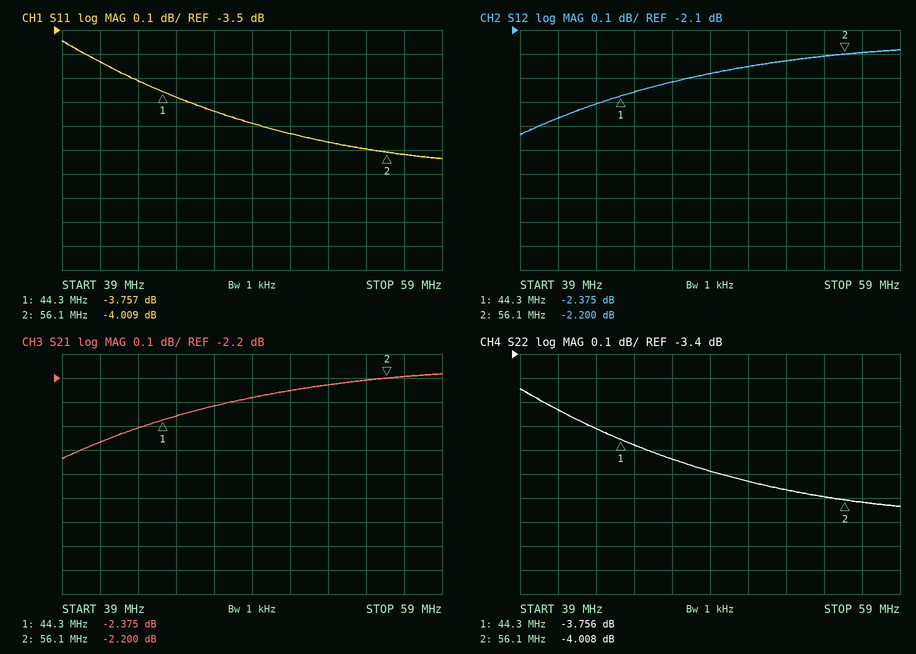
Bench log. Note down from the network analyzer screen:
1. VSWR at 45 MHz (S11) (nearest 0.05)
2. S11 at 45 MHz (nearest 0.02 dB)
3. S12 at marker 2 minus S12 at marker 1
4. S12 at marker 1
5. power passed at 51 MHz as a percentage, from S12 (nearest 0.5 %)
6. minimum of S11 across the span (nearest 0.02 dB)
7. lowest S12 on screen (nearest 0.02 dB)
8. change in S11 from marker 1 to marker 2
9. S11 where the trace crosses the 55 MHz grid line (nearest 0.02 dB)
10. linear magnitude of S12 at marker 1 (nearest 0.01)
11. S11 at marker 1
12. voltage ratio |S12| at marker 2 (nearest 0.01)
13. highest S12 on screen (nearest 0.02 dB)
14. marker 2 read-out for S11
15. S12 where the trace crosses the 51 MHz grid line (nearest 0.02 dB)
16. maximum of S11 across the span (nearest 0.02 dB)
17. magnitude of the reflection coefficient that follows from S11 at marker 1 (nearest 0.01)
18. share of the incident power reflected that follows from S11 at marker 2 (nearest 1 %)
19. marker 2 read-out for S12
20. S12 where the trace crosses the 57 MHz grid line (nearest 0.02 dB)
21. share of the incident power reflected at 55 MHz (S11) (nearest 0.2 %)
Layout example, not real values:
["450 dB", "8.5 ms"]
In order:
["4.65", "-3.78 dB", "0.175 dB", "-2.375 dB", "59.5 %", "-4.04 dB", "-2.54 dB", "-0.252 dB", "-4.00 dB", "0.76", "-3.757 dB", "0.78", "-2.18 dB", "-4.009 dB", "-2.26 dB", "-3.54 dB", "0.65", "40 %", "-2.200 dB", "-2.20 dB", "39.8 %"]
